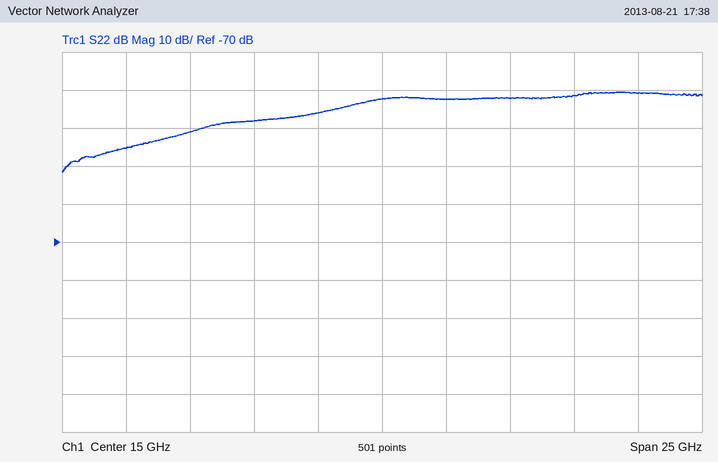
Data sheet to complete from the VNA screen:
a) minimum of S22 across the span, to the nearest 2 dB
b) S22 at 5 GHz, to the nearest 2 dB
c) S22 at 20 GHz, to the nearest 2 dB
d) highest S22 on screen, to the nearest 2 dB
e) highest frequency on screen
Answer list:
-52 dB
-46 dB
-32 dB
-30 dB
27.5 GHz
